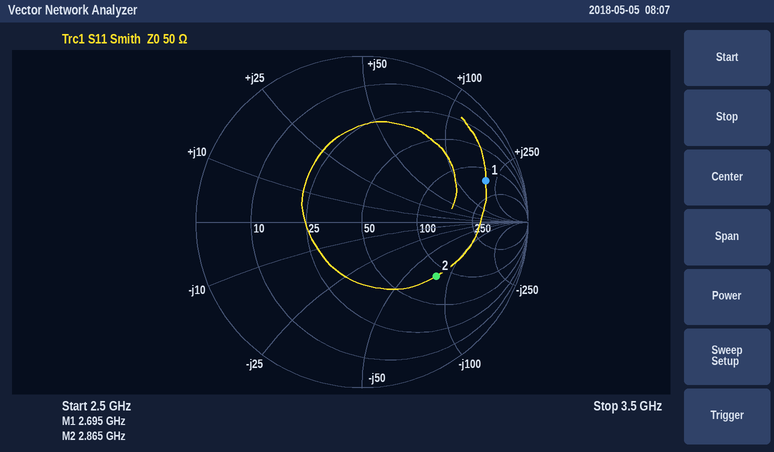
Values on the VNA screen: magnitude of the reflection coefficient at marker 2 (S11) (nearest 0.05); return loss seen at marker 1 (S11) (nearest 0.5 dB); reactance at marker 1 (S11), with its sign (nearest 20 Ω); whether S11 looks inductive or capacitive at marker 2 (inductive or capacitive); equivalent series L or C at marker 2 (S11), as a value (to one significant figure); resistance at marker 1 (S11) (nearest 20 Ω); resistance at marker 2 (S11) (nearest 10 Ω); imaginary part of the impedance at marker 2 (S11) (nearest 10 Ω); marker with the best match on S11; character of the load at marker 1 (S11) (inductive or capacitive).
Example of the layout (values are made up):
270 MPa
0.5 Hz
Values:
0.55
2.0 dB
+200 Ω
capacitive
700 fF
160 Ω
80 Ω
-80 Ω
marker 2
inductive
